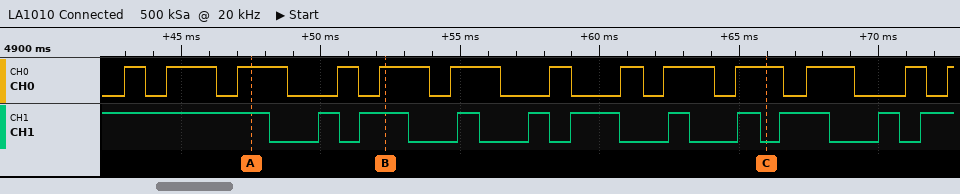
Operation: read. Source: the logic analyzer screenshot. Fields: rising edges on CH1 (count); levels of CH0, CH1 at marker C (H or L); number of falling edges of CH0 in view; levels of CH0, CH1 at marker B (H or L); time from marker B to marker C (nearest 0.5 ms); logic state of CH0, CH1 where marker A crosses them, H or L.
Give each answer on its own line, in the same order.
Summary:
10
CH0=H, CH1=L
12
CH0=H, CH1=H
13.5 ms
CH0=H, CH1=H
